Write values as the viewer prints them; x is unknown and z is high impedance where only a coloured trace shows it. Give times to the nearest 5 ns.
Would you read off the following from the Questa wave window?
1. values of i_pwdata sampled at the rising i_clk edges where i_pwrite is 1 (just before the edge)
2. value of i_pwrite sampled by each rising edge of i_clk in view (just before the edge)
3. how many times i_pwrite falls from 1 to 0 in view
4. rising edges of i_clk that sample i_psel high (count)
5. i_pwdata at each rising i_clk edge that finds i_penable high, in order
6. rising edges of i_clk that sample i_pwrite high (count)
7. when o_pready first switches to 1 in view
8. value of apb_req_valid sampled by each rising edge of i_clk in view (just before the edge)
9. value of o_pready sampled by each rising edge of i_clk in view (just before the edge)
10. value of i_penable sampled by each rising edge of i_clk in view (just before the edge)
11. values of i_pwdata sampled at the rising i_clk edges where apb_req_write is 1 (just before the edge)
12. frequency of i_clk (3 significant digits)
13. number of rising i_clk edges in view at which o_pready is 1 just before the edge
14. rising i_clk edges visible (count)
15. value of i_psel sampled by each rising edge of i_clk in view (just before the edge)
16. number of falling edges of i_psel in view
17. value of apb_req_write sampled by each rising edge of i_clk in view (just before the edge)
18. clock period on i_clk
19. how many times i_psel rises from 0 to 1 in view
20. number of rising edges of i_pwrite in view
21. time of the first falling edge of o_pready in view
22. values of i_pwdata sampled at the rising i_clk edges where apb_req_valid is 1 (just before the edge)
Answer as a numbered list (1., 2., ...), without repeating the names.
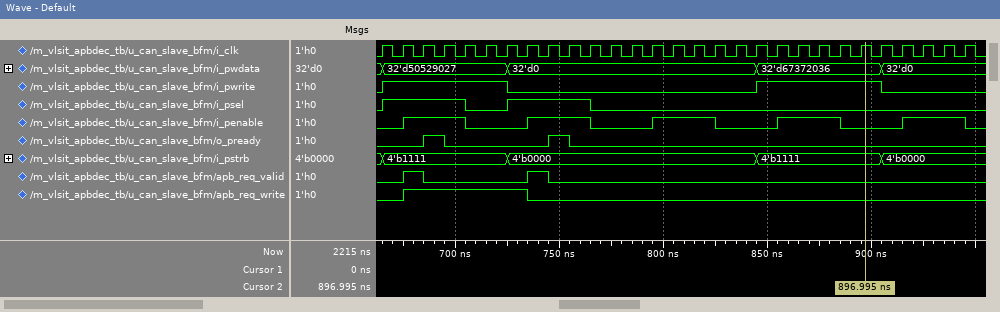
1. 32'd50529027, 32'd50529027, 32'd50529027, 32'd50529027, 32'd50529027, 32'd50529027, 32'd67372036, 32'd67372036, 32'd67372036, 32'd67372036, 32'd67372036, 32'd67372036
2. 0 1 1 1 1 1 1 0 0 0 0 0 0 0 0 0 0 0 0 1 1 1 1 1 1 0 0 0 0
3. 2
4. 8
5. 32'd50529027, 32'd50529027, 32'd50529027, 32'd0, 32'd0, 32'd0, 32'd0, 32'd0, 32'd0, 32'd67372036, 32'd67372036, 32'd67372036, 32'd0, 32'd0, 32'd0
6. 12
7. 685 ns
8. 0 0 1 0 0 0 0 0 1 0 0 0 0 0 0 0 0 0 0 0 0 0 0 0 0 0 0 0 0
9. 0 0 0 1 0 0 0 0 0 1 0 0 0 0 0 0 0 0 0 0 0 0 0 0 0 0 0 0 0
10. 0 0 1 1 1 0 0 0 1 1 1 0 0 0 1 1 1 0 0 0 1 1 1 0 0 0 1 1 1
11. 32'd50529027, 32'd50529027, 32'd50529027, 32'd50529027, 32'd50529027, 32'd0
12. 100 MHz
13. 2
14. 29
15. 0 1 1 1 1 0 0 1 1 1 1 0 0 0 0 0 0 0 0 0 0 0 0 0 0 0 0 0 0
16. 2
17. 0 0 1 1 1 1 1 1 0 0 0 0 0 0 0 0 0 0 0 0 0 0 0 0 0 0 0 0 0
18. 10 ns
19. 2
20. 2
21. 695 ns
22. 32'd50529027, 32'd0
